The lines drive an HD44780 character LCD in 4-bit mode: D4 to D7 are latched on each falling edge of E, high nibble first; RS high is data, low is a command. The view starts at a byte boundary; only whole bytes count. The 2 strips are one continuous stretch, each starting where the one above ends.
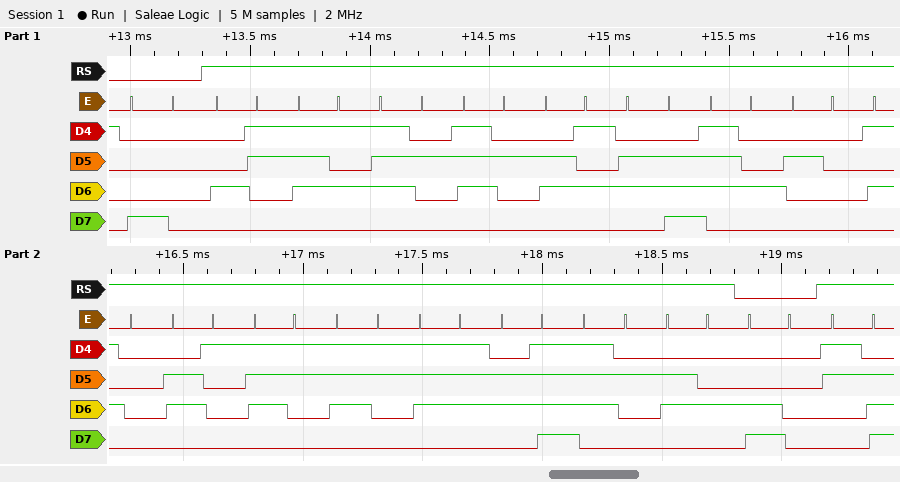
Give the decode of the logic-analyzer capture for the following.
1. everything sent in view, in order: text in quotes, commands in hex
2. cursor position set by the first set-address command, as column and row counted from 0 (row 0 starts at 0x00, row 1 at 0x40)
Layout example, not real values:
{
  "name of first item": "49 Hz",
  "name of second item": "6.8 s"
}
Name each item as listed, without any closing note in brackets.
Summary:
{
  "everything sent in view, in order: text in quotes, commands in hex": "0x80 \"Current Password\" 0xC0 \">\"",
  "cursor position set by the first set-address command, as column and row counted from 0": "column 0, row 0"
}
